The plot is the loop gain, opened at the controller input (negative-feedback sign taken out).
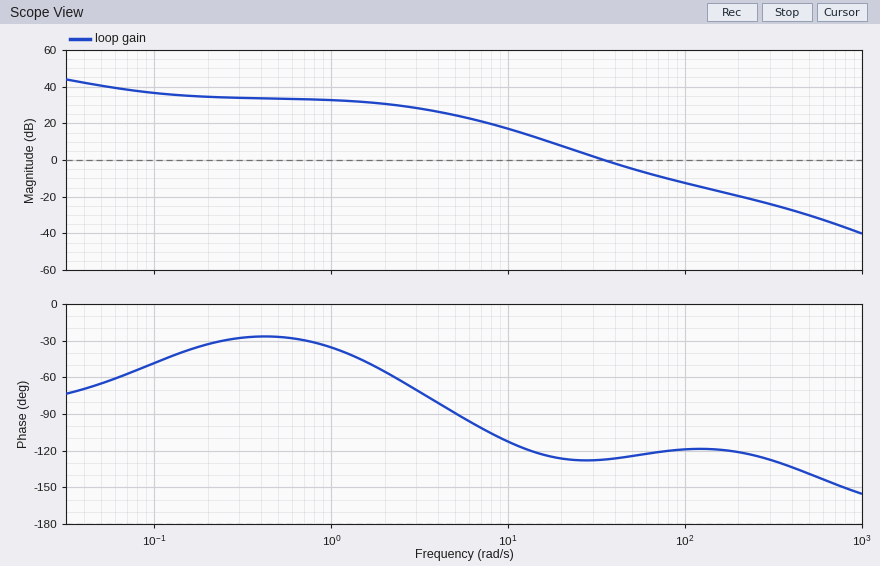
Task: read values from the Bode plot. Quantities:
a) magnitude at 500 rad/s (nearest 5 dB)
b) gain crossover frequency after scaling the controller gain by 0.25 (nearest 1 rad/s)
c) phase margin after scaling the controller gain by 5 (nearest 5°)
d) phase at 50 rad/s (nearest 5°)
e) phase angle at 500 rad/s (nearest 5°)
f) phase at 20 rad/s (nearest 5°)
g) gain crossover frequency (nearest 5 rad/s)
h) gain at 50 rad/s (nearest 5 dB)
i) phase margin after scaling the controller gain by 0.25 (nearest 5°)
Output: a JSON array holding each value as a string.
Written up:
["-30 dB", "15 rad/s", "60°", "-125°", "-140°", "-125°", "35 rad/s", "-5 dB", "60°"]
